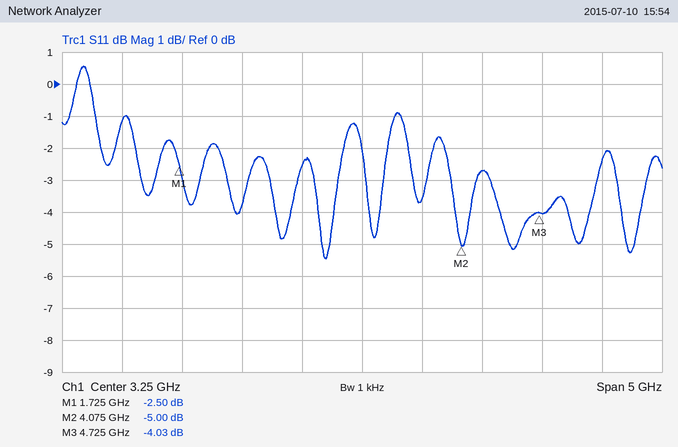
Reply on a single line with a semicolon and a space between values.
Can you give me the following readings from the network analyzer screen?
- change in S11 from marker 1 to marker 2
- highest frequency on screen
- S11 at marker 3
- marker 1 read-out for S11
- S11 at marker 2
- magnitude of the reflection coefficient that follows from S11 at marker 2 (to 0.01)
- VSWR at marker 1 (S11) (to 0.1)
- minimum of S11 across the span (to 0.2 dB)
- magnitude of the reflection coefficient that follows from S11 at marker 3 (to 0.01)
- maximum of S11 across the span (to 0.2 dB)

-2.50 dB; 5.75 GHz; -4.03 dB; -2.50 dB; -5.00 dB; 0.56; 7.0; -5.4 dB; 0.63; 0.6 dB
